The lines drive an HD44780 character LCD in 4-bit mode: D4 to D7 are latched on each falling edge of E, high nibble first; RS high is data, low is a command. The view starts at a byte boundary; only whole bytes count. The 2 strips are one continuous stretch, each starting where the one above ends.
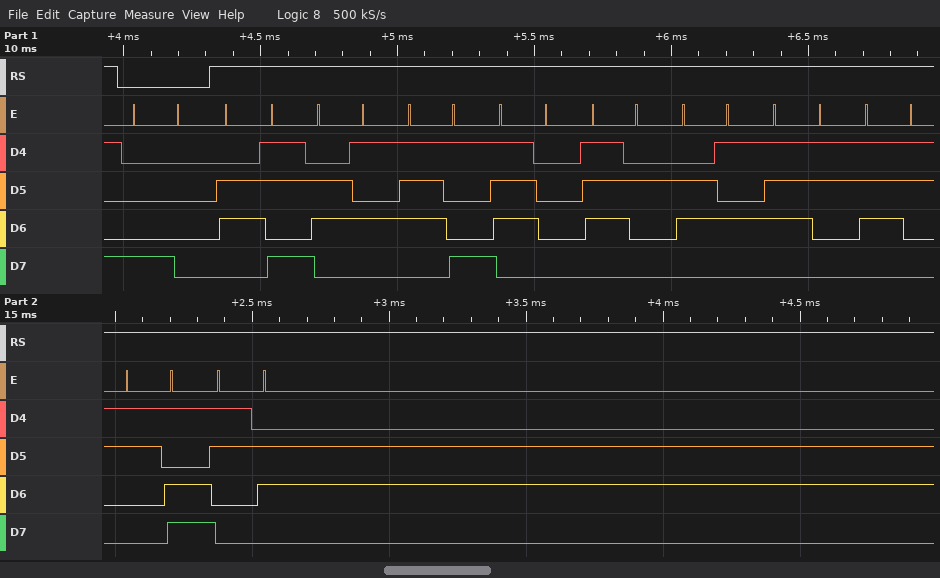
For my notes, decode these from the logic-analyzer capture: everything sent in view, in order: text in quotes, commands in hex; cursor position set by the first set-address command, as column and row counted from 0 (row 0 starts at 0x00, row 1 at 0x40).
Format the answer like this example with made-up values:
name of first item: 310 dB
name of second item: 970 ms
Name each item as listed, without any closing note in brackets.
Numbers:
everything sent in view, in order: text in quotes, commands in hex: 0x80 "keypress=6"
cursor position set by the first set-address command, as column and row counted from 0: column 0, row 0
